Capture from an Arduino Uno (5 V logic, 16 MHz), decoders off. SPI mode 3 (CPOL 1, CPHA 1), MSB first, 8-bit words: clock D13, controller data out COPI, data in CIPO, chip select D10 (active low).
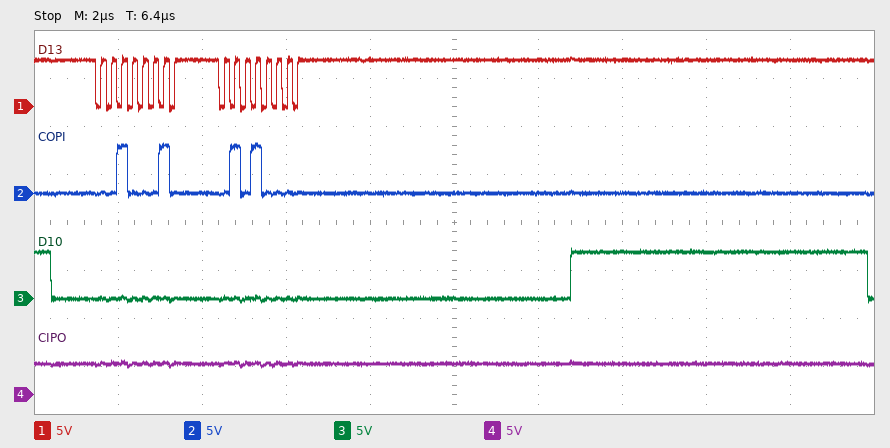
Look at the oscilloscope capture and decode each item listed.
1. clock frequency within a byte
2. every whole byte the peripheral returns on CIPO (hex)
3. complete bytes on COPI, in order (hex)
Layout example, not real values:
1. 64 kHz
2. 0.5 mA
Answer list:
1. 4 MHz
2. FF FF
3. 22 50
